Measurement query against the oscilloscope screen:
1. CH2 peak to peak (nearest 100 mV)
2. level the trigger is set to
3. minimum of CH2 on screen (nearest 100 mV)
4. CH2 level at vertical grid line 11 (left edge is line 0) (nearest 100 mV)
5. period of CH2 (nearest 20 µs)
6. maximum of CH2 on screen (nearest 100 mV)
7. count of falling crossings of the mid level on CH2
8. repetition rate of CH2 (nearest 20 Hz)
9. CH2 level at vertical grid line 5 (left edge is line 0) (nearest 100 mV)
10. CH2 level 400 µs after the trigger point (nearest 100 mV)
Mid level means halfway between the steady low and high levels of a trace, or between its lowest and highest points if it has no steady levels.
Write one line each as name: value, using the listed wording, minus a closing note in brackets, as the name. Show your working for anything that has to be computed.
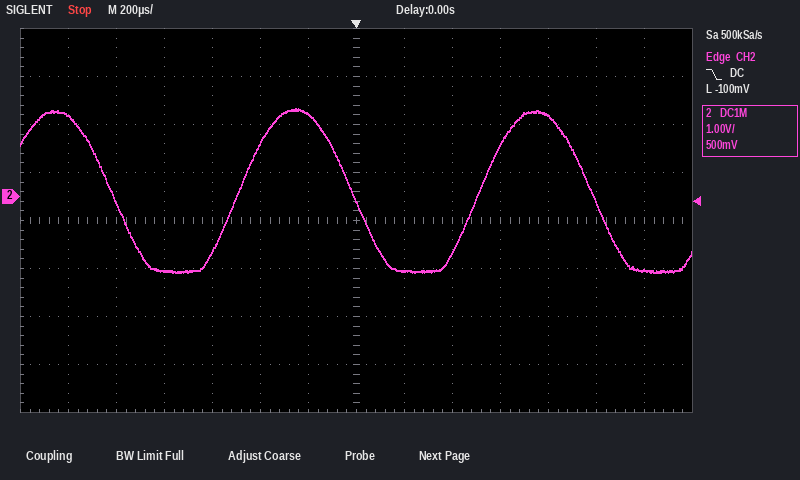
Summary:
CH2 peak to peak: 1.8 V − (-1.6 V) = 3.4 V
level the trigger is set to: -100 mV
minimum of CH2 on screen: -1.6 V
CH2 level at vertical grid line 11 (left edge is line 0): 1.7 V
period of CH2: 1.00 ms
maximum of CH2 on screen: 1.8 V
count of falling crossings of the mid level on CH2: 3
repetition rate of CH2: 1 / 1.00 ms ≈ 1.00 kHz
CH2 level at vertical grid line 5 (left edge is line 0): 1.1 V
CH2 level 400 µs after the trigger point: -1.2 V
